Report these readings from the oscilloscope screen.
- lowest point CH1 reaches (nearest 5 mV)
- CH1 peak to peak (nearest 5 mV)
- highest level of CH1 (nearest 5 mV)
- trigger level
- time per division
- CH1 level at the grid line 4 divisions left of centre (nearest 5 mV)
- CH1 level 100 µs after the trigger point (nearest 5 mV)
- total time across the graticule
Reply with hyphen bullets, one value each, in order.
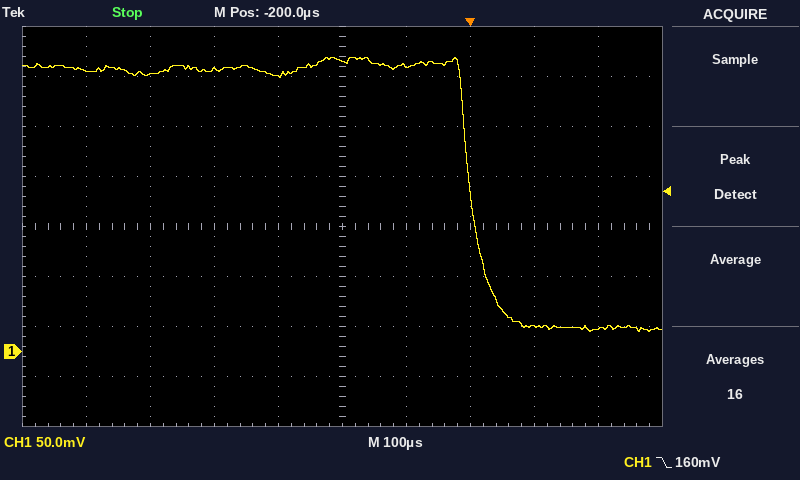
- 20 mV
- 275 mV
- 295 mV
- 160 mV
- 100 µs
- 280 mV
- 25 mV
- 1 ms
